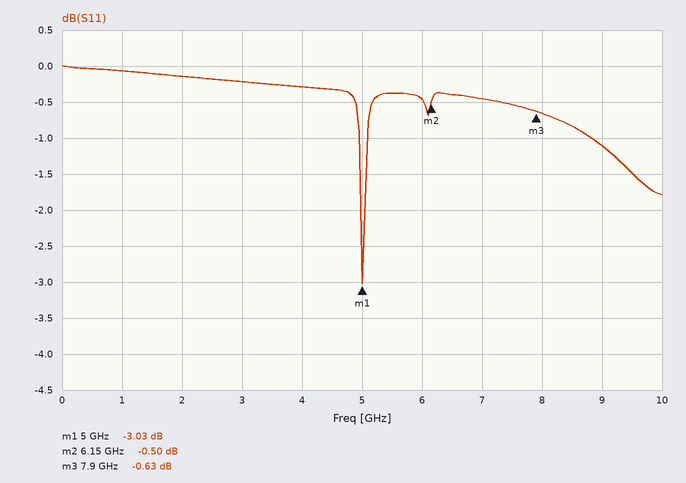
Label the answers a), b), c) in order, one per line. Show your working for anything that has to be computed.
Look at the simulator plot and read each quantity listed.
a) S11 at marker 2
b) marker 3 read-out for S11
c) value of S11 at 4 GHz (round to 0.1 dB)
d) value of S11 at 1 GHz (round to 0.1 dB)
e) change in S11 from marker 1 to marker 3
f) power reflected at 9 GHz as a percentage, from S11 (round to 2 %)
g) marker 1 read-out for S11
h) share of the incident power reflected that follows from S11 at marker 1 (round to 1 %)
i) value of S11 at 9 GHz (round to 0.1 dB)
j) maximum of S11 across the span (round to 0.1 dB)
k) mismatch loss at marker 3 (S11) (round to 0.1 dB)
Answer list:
a) -0.50 dB
b) -0.63 dB
c) -0.3 dB
d) -0.1 dB
e) -0.63 − (-3.03) = 2.40 dB
f) 10^(-1.1/10) ≈ 78 %
g) -3.03 dB
h) 10^(-3.03/10) ≈ 50 %
i) -1.1 dB
j) 0.0 dB
k) −10 log10(1 − 10^(-0.63/10)) ≈ 8.7 dB
